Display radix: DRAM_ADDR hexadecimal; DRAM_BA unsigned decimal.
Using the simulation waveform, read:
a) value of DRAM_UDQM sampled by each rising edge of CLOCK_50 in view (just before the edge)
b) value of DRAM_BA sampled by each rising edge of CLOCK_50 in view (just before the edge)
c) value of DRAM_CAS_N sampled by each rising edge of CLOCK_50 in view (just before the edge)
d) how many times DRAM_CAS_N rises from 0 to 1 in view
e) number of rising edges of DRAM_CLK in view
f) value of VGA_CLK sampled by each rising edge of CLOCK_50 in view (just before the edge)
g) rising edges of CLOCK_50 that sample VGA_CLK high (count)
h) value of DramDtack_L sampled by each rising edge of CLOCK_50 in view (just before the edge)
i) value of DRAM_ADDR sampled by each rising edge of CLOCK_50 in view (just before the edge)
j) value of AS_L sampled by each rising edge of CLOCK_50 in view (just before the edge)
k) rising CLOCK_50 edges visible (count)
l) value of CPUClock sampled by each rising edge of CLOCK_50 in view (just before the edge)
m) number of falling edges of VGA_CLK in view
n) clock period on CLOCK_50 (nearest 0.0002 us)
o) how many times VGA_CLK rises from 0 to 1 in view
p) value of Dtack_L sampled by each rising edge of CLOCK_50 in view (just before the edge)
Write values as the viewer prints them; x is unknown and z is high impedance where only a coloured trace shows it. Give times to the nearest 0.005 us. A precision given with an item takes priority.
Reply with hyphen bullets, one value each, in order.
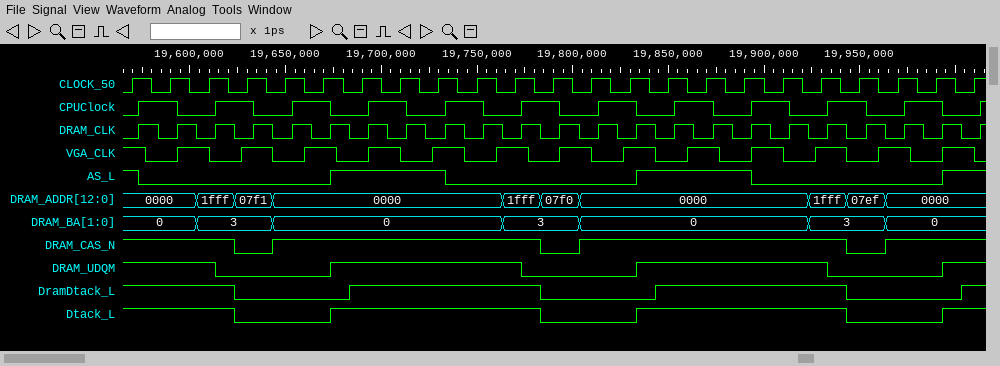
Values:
- 1 1 1 0 0 0 1 1 1 1 1 0 0 0 1 1 1 1 1 0 0 0 1
- 0, 0, 3, 3, 0, 0, 0, 0, 0, 0, 3, 3, 0, 0, 0, 0, 0, 0, 3, 3, 0, 0, 0
- 1 1 1 0 1 1 1 1 1 1 1 0 1 1 1 1 1 1 1 0 1 1 1
- 3
- 23
- 1 0 1 1 0 1 0 1 1 0 1 0 1 1 0 1 0 1 1 0 1 0 1
- 14
- 1 1 1 0 0 0 1 1 1 1 1 0 0 0 1 1 1 1 1 0 0 0 1
- 0000, 0000, 1fff, 07f1, 0000, 0000, 0000, 0000, 0000, 0000, 1fff, 07f0, 0000, 0000, 0000, 0000, 0000, 0000, 1fff, 07ef, 0000, 0000, 0000
- 1 0 0 0 0 0 1 1 1 0 0 0 0 0 1 1 1 0 0 0 0 0 1
- 23
- 0 1 0 1 0 1 0 1 0 1 0 1 0 1 0 1 0 1 0 1 0 1 0
- 14
- 0.02 us
- 13
- 1 1 1 0 0 0 1 1 1 1 1 0 0 0 1 1 1 1 1 0 0 0 1
